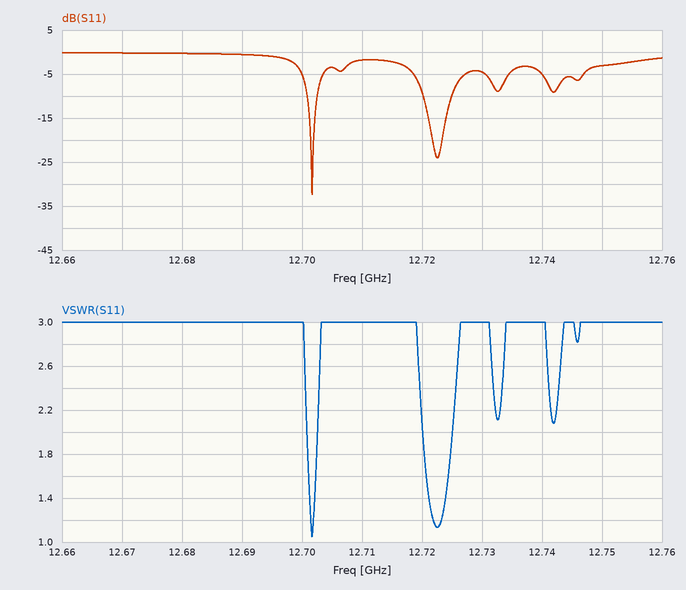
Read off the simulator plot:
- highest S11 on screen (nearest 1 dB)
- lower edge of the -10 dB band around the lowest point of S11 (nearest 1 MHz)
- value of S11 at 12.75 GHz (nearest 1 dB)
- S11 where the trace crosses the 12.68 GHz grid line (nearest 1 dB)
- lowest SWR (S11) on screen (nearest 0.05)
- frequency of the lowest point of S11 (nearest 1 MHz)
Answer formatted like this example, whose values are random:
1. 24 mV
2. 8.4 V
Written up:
1. 0 dB
2. 12.701 GHz
3. -3 dB
4. 0 dB
5. 1.05
6. 12.702 GHz
